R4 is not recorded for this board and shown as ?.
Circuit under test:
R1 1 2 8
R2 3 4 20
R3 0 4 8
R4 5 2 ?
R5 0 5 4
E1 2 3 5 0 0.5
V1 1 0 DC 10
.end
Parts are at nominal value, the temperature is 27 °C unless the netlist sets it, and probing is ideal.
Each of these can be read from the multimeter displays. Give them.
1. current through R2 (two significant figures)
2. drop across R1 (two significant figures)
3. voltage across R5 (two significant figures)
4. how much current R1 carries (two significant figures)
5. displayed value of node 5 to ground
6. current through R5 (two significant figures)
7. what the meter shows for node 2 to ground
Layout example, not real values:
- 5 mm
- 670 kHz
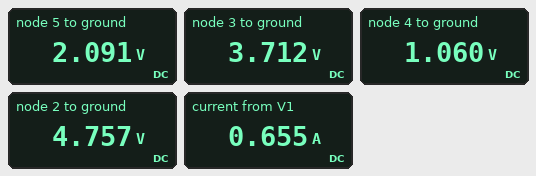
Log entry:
- 130 mA
- 5.2 V
- 2.1 V
- 660 mA
- 2.091 V
- 520 mA
- 4.757 V
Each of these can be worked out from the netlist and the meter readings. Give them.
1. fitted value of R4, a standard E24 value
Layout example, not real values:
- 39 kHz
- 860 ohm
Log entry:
- 5.1 Ω
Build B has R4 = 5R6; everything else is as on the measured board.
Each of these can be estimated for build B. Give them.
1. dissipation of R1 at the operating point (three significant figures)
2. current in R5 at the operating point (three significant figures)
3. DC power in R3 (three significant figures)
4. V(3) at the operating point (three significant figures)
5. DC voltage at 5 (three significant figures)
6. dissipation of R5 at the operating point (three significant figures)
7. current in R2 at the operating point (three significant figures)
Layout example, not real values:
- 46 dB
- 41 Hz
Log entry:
- 3.31 W
- 506 mA
- 151 mW
- 3.84 V
- 2.02 V
- 1.02 W
- 137 mA
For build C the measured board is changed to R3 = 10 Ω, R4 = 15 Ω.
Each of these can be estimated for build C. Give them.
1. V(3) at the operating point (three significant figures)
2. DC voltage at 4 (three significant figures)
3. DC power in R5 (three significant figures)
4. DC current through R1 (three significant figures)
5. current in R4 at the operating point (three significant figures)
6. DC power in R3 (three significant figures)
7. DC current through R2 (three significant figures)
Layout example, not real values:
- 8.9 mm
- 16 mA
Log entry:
- 5.39 V
- 1.80 V
- 402 mW
- 497 mA
- 317 mA
- 323 mW
- 180 mA
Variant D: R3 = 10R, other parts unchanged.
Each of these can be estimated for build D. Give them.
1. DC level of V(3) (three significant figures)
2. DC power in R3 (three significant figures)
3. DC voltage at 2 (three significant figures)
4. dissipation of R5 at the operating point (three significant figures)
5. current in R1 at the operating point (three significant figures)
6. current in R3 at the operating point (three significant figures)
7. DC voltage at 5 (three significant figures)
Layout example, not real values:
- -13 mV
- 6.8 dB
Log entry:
- 3.74 V
- 155 mW
- 4.79 V
- 1.11 W
- 651 mA
- 125 mA
- 2.11 V
